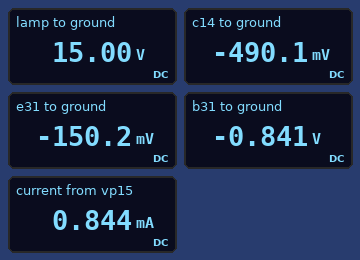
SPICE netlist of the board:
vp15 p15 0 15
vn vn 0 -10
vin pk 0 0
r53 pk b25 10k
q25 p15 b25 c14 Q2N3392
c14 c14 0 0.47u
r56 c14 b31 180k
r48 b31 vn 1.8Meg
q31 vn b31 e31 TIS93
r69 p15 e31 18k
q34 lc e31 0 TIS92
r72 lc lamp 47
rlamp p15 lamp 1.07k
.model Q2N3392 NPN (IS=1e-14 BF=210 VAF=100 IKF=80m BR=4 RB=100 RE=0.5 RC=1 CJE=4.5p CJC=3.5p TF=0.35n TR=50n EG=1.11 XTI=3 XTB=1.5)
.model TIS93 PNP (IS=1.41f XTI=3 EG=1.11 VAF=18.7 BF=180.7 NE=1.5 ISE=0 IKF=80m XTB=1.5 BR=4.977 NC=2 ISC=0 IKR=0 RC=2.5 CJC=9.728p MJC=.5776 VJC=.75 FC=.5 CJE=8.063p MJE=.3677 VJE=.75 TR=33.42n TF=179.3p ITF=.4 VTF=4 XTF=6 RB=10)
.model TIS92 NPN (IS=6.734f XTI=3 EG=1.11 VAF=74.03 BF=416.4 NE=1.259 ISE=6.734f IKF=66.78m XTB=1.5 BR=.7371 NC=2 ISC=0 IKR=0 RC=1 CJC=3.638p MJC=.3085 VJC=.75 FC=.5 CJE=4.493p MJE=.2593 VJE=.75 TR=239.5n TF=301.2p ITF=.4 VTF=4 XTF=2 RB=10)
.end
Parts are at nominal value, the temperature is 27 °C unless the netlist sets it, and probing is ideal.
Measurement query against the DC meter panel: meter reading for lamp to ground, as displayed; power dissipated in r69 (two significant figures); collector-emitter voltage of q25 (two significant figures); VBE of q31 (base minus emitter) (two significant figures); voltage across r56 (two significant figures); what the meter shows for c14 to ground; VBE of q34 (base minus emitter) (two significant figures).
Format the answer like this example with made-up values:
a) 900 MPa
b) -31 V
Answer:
a) 15.00 V
b) 13 mW
c) 15 V
d) -690 mV
e) 350 mV
f) -490.1 mV
g) -150 mV
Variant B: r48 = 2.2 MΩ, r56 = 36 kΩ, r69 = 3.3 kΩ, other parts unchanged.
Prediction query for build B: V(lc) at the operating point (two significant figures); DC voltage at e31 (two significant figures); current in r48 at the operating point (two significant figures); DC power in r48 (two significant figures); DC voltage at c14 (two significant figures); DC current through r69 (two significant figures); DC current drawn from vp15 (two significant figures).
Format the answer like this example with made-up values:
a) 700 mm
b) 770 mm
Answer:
a) 75 mV
b) 780 mV
c) 4.6 µA
d) 46 µW
e) 76 mV
f) 4.3 mA
g) 18 mA
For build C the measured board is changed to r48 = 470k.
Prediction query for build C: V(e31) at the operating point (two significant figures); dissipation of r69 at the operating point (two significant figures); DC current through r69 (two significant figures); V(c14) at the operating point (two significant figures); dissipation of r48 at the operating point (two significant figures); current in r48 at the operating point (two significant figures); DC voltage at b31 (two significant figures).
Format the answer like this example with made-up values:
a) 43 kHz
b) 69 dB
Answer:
a) -2.0 V
b) 16 mW
c) 940 µA
d) -540 mV
e) 110 µW
f) 16 µA
g) -2.7 V
